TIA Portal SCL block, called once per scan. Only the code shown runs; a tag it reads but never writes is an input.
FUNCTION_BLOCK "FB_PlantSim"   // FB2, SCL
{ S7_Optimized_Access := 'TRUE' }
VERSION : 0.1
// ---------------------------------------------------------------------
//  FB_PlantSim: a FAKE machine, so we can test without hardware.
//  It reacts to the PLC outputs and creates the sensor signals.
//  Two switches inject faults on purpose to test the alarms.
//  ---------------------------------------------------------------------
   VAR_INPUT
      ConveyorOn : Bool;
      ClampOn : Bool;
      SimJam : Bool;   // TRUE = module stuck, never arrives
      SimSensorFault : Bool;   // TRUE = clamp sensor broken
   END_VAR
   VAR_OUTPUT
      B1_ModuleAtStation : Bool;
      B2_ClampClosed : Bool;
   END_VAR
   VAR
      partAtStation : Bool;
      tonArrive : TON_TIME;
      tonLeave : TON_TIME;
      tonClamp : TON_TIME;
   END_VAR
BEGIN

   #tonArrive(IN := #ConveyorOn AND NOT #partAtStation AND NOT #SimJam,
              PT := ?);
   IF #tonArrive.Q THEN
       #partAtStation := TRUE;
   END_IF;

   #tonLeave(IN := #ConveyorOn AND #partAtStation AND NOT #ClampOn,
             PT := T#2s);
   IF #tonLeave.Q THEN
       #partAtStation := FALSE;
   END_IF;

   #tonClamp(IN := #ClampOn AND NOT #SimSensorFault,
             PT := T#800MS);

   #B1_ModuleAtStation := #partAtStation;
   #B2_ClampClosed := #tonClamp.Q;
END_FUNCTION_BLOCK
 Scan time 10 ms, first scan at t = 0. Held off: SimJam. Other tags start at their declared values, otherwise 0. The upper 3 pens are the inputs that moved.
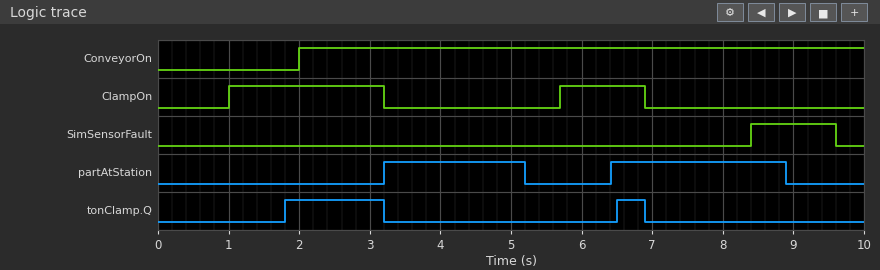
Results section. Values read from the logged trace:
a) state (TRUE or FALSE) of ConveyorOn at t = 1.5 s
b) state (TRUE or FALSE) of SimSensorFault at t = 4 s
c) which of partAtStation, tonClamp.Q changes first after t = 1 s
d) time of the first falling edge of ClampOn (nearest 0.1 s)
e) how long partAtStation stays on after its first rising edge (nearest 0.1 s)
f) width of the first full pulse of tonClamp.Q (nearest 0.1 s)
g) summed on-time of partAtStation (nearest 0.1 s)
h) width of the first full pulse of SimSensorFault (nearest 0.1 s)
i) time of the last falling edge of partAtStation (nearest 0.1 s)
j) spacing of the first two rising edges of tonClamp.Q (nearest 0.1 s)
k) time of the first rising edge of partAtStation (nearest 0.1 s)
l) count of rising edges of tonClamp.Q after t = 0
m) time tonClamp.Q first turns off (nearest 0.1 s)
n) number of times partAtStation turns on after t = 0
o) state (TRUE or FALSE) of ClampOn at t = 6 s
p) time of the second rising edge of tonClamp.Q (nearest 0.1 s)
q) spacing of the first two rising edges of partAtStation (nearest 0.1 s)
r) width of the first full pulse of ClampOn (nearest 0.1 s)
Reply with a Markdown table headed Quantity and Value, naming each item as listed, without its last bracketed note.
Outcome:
| Quantity | Value |
|---|---|
| state (TRUE or FALSE) of ConveyorOn at t = 1.5 s | FALSE |
| state (TRUE or FALSE) of SimSensorFault at t = 4 s | FALSE |
| which of partAtStation, tonClamp.Q changes first after t = 1 s | tonClamp.Q |
| time of the first falling edge of ClampOn | 3.2 s |
| how long partAtStation stays on after its first rising edge | 2.0 s |
| width of the first full pulse of tonClamp.Q | 1.4 s |
| summed on-time of partAtStation | 4.5 s |
| width of the first full pulse of SimSensorFault | 1.2 s |
| time of the last falling edge of partAtStation | 8.9 s |
| spacing of the first two rising edges of tonClamp.Q | 4.7 s |
| time of the first rising edge of partAtStation | 3.2 s |
| count of rising edges of tonClamp.Q after t = 0 | 2 |
| time tonClamp.Q first turns off | 3.2 s |
| number of times partAtStation turns on after t = 0 | 2 |
| state (TRUE or FALSE) of ClampOn at t = 6 s | TRUE |
| time of the second rising edge of tonClamp.Q | 6.5 s |
| spacing of the first two rising edges of partAtStation | 3.2 s |
| width of the first full pulse of ClampOn | 2.2 s |
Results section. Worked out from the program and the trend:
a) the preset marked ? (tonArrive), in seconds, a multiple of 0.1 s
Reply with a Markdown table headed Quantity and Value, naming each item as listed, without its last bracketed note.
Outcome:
| Quantity | Value |
|---|---|
| the preset marked ? (tonArrive), in seconds, a multiple of 0.1 s | 1.2 s |
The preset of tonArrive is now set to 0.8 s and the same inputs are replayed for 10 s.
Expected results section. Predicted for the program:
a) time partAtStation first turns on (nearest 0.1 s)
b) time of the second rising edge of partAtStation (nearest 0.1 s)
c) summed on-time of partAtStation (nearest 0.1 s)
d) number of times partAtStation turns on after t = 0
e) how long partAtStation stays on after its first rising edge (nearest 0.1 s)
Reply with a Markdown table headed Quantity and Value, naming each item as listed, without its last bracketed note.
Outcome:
| Quantity | Value |
|---|---|
| time partAtStation first turns on | 2.8 s |
| time of the second rising edge of partAtStation | 6.0 s |
| summed on-time of partAtStation | 5.6 s |
| number of times partAtStation turns on after t = 0 | 3 |
| how long partAtStation stays on after its first rising edge | 2.4 s |
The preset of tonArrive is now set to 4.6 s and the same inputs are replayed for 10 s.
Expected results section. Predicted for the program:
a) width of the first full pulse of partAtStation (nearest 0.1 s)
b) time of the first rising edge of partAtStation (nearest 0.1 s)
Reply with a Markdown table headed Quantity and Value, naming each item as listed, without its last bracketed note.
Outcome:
| Quantity | Value |
|---|---|
| width of the first full pulse of partAtStation | 2.3 s |
| time of the first rising edge of partAtStation | 6.6 s |
